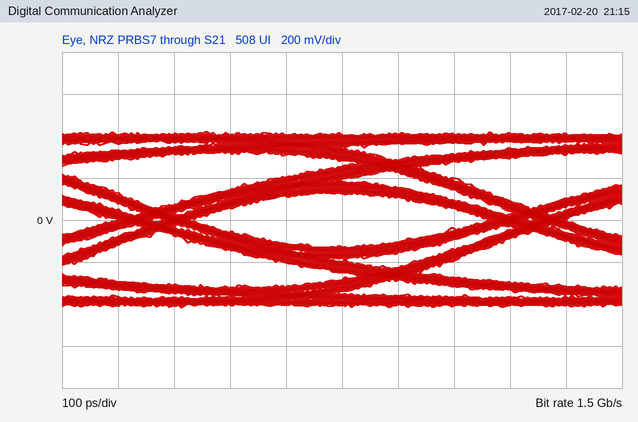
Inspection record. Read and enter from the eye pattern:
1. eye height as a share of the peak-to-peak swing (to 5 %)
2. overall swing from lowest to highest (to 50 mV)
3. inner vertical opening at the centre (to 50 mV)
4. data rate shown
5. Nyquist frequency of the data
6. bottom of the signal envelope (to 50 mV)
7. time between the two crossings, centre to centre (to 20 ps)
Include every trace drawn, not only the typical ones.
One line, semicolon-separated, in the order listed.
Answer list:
30 %; 850 mV; 250 mV; 1.5 Gb/s; 750 MHz; -400 mV; 660 ps
